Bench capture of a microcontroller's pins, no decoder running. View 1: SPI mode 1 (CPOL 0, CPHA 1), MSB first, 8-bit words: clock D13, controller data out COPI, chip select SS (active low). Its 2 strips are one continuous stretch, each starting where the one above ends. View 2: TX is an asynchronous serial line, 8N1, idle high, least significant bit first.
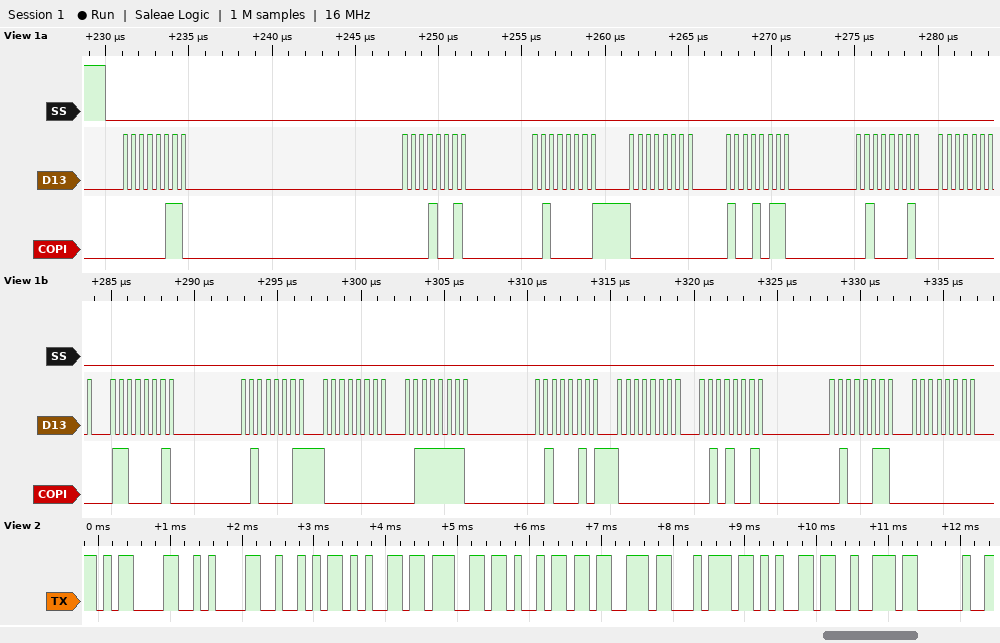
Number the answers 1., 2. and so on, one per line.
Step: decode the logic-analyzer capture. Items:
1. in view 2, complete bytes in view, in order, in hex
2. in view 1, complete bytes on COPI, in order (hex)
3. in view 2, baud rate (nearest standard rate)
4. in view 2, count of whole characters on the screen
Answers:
1. 0D 0A 52 65 67 69 73 74 65 72 20
2. 06 12 41 00 96 42 00 C2 43 00 7E 45 00 52 46 00
3. 9600 baud
4. 11
